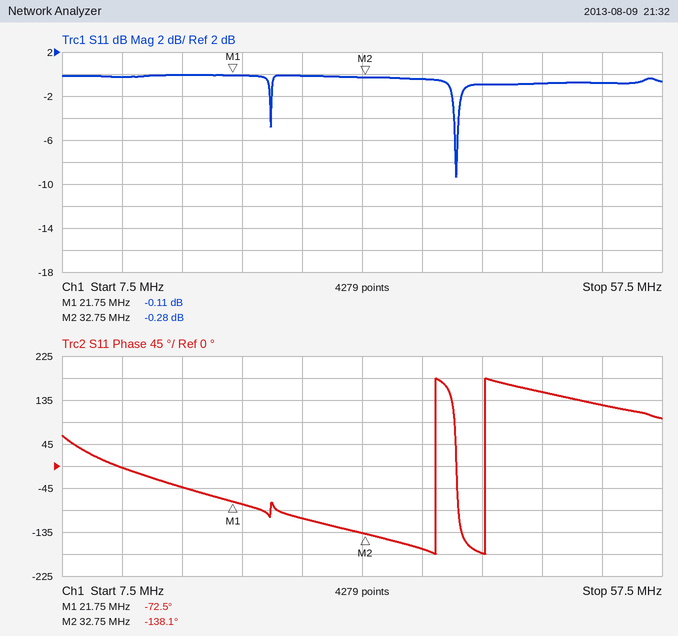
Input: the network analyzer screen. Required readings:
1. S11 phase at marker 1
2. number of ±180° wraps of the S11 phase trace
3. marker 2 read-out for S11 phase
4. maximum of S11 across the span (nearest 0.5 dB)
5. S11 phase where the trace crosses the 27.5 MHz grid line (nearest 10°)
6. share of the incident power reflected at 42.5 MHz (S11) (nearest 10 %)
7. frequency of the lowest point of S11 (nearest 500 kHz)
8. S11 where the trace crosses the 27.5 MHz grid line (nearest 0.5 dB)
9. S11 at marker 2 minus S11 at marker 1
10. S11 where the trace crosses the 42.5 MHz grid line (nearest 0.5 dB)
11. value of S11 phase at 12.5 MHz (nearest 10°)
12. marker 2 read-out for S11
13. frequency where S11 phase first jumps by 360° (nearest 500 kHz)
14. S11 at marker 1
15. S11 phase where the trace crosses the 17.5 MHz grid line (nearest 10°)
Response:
-72.5°
2
-138.1°
0.0 dB
-110°
80 %
40.5 MHz
0.0 dB
-0.17 dB
-1.0 dB
0°
-0.28 dB
38.5 MHz
-0.11 dB
-40°
